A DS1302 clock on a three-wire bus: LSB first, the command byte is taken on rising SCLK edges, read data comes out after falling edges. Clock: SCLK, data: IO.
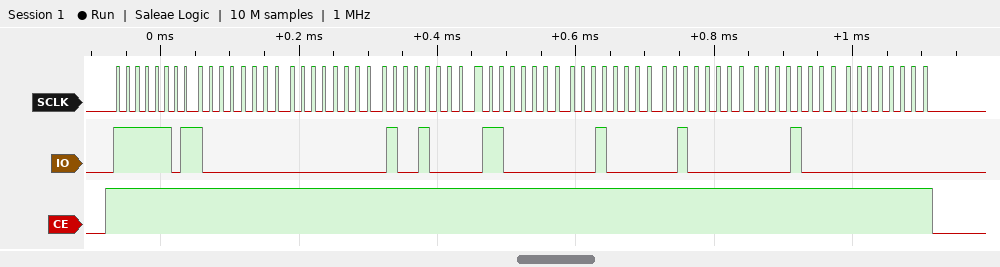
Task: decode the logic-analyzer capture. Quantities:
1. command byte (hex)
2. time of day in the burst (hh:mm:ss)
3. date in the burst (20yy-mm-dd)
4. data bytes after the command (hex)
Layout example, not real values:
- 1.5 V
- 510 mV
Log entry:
- 0xBF
- 12:00:01
- 2010-08-06
- 01 00 12 06 08 04 10 00
